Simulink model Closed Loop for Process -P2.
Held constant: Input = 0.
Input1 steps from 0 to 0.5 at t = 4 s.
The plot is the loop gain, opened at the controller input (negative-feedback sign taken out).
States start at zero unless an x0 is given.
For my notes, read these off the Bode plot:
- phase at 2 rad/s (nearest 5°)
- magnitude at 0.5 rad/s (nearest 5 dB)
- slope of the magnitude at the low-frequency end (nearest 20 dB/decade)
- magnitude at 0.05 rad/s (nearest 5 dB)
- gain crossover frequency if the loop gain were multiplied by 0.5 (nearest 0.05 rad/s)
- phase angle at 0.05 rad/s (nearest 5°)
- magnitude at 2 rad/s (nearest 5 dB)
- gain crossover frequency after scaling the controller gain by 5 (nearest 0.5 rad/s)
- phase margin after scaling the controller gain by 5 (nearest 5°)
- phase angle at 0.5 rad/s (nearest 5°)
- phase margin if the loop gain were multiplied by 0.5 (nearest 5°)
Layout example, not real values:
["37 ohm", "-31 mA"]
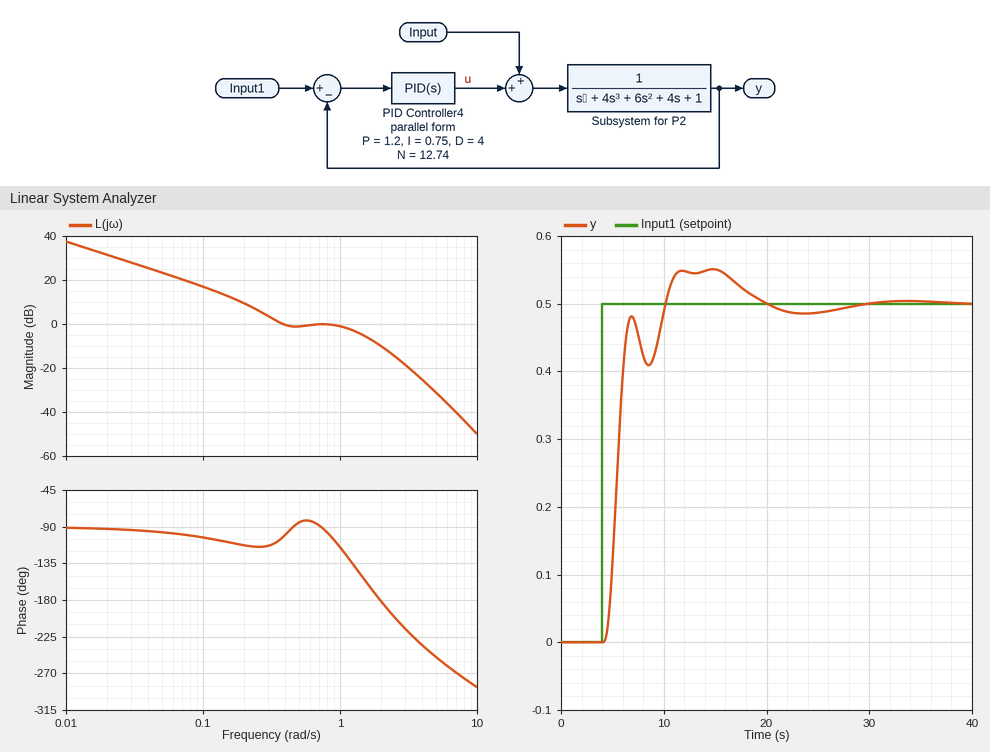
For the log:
["-180°", "0 dB", "-20 dB/decade", "25 dB", "0.25 rad/s", "-95°", "-10 dB", "2.5 rad/s", "-20°", "-85°", "65°"]
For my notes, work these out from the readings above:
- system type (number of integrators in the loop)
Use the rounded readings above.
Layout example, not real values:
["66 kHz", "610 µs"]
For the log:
["1"]
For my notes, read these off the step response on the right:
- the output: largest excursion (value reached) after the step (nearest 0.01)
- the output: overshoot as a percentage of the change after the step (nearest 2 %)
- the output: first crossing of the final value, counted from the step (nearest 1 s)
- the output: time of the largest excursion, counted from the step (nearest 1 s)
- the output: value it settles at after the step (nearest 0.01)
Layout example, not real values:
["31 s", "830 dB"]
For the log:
["0.55", "10 %", "6 s", "11 s", "0.50"]
